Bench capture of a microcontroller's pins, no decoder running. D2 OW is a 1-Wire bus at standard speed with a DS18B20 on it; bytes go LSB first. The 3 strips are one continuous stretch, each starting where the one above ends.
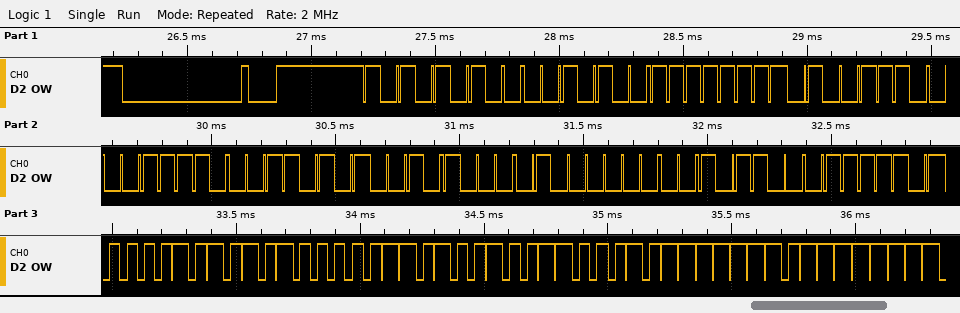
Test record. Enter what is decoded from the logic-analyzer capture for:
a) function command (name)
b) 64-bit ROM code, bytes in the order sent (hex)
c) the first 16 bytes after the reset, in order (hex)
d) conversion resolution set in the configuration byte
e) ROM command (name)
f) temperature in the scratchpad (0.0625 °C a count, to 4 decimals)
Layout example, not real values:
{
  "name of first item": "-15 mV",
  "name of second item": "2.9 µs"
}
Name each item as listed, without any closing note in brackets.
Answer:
{
  "function command": "Read Scratchpad",
  "64-bit ROM code, bytes in the order sent": "28 FF 72 78 AC 14 02 34",
  "the first 16 bytes after the reset, in order": "55 28 FF 72 78 AC 14 02 34 BE 50 05 4B 46 7F FF",
  "conversion resolution set in the configuration byte": "12 bits",
  "ROM command": "Match ROM",
  "temperature in the scratchpad": "85.0000 °C"
}
